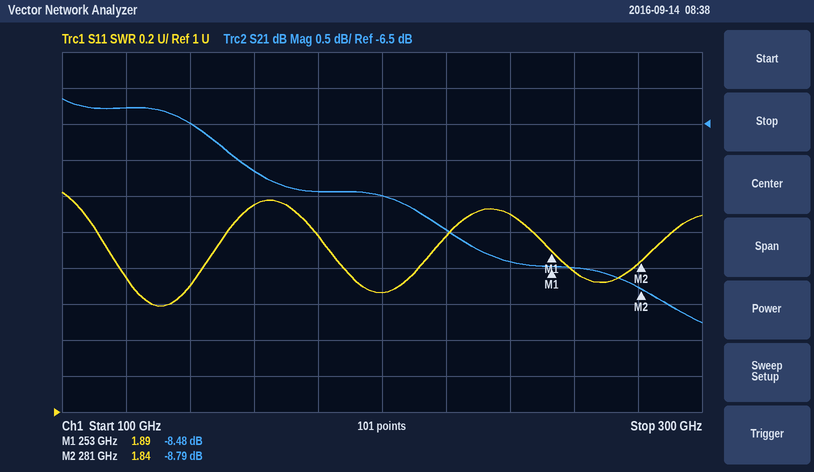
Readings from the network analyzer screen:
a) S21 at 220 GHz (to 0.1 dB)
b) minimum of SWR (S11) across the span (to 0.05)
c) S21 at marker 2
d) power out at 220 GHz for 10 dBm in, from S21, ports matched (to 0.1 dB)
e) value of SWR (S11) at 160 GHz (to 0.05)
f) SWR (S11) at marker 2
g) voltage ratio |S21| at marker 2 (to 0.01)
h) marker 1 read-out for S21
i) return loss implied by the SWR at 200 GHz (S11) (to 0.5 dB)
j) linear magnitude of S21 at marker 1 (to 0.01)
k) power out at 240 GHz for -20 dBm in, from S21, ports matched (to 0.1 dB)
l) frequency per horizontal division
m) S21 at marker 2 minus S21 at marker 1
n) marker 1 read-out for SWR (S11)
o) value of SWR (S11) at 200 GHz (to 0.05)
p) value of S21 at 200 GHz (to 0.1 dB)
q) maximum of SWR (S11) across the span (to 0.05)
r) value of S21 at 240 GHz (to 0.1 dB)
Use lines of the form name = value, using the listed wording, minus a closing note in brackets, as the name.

S21 at 220 GHz = -8.0 dB
minimum of SWR (S11) across the span = 1.60
S21 at marker 2 = -8.79 dB
power out at 220 GHz for 10 dBm in, from S21, ports matched = 2.0 dBm
value of SWR (S11) at 160 GHz = 2.15
SWR (S11) at marker 2 = 1.84
voltage ratio |S21| at marker 2 = 0.36
marker 1 read-out for S21 = -8.48 dB
return loss implied by the SWR at 200 GHz (S11) = 12.0 dB
linear magnitude of S21 at marker 1 = 0.38
power out at 240 GHz for -20 dBm in, from S21, ports matched = -28.4 dBm
frequency per horizontal division = 20 GHz
S21 at marker 2 minus S21 at marker 1 = -0.31 dB
marker 1 read-out for SWR = 1.89
value of SWR (S11) at 200 GHz = 1.65
value of S21 at 200 GHz = -7.5 dB
maximum of SWR (S11) across the span = 2.20
value of S21 at 240 GHz = -8.4 dB
